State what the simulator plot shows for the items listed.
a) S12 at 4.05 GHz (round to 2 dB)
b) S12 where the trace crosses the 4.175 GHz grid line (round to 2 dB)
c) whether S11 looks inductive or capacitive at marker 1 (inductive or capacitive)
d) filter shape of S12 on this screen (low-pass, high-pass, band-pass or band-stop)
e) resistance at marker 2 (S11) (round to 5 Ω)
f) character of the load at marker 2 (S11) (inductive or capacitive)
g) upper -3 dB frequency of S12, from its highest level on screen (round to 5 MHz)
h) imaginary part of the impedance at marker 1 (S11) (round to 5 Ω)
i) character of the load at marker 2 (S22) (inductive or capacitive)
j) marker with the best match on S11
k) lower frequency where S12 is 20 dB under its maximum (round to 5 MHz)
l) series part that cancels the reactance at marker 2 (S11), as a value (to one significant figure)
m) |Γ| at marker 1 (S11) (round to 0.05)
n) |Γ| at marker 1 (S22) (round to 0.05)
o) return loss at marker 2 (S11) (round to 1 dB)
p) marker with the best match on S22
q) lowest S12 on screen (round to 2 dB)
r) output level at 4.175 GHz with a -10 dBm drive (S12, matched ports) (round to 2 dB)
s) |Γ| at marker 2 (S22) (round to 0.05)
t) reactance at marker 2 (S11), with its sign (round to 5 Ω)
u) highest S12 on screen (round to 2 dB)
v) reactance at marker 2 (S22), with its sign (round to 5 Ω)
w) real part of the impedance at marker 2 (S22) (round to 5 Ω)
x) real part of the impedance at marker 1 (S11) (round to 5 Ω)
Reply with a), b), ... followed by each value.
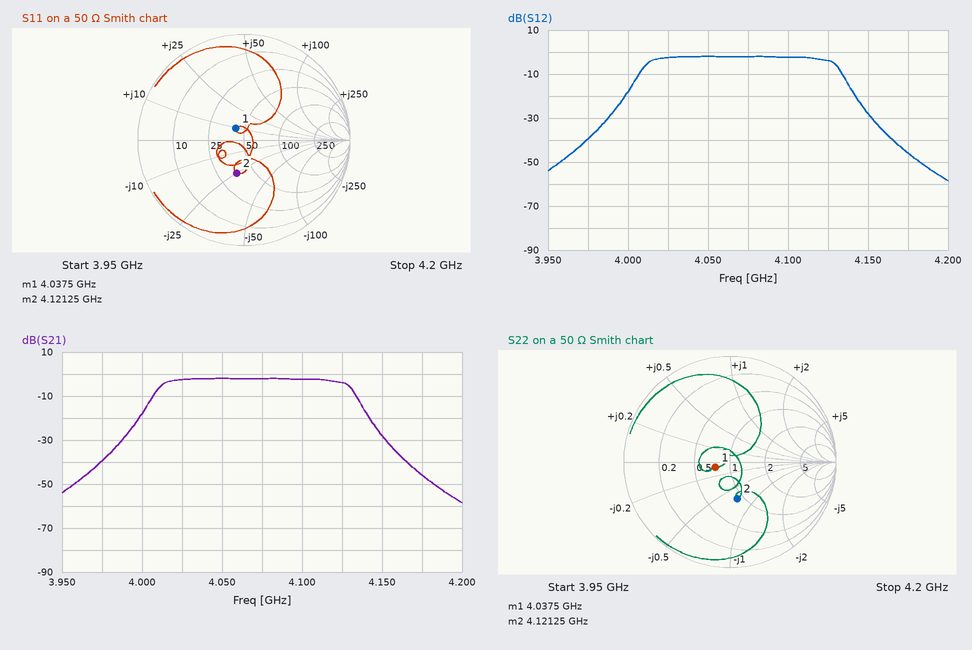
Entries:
a) -2 dB
b) -46 dB
c) inductive
d) band-pass
e) 35 Ω
f) capacitive
g) 4.130 GHz
h) +10 Ω
i) capacitive
j) marker 1
k) 3.995 GHz
l) 1.0 nH
m) 0.15
n) 0.15
o) 10 dB
p) marker 1
q) -58 dB
r) -56 dBm
s) 0.35
t) -25 Ω
u) -2 dB
v) -35 Ω
w) 45 Ω
x) 40 Ω
